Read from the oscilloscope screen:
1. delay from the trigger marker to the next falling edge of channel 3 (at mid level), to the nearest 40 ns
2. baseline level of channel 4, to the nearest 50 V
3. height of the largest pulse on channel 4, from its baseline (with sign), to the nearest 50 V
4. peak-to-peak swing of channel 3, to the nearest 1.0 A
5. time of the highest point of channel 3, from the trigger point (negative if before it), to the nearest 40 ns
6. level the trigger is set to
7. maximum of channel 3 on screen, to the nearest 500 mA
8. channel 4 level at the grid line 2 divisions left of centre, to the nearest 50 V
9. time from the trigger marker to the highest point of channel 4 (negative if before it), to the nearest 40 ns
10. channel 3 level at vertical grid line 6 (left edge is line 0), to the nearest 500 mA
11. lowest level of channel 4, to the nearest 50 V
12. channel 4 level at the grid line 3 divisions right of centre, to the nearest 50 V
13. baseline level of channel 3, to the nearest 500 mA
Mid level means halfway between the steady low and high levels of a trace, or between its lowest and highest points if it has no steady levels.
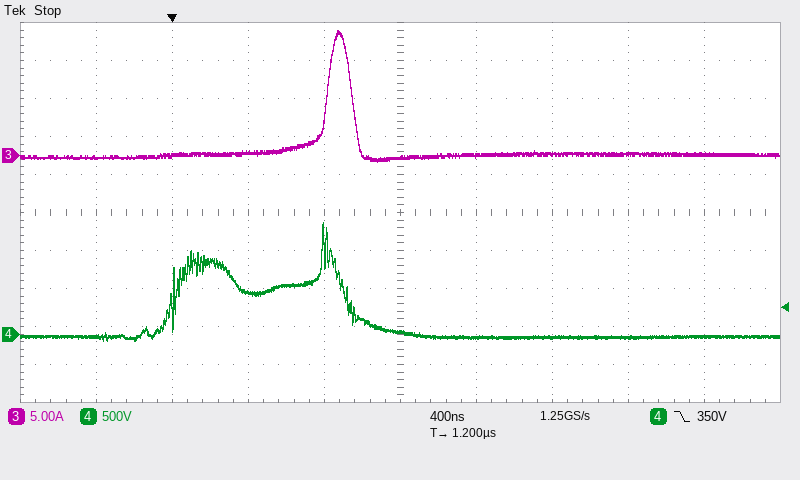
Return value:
960 ns
-50 V
+1.50 kV
17.0 A
+880 ns
350 V
16.5 A
550 V
+800 ns
0.0 A
-100 V
-50 V
0.0 A
